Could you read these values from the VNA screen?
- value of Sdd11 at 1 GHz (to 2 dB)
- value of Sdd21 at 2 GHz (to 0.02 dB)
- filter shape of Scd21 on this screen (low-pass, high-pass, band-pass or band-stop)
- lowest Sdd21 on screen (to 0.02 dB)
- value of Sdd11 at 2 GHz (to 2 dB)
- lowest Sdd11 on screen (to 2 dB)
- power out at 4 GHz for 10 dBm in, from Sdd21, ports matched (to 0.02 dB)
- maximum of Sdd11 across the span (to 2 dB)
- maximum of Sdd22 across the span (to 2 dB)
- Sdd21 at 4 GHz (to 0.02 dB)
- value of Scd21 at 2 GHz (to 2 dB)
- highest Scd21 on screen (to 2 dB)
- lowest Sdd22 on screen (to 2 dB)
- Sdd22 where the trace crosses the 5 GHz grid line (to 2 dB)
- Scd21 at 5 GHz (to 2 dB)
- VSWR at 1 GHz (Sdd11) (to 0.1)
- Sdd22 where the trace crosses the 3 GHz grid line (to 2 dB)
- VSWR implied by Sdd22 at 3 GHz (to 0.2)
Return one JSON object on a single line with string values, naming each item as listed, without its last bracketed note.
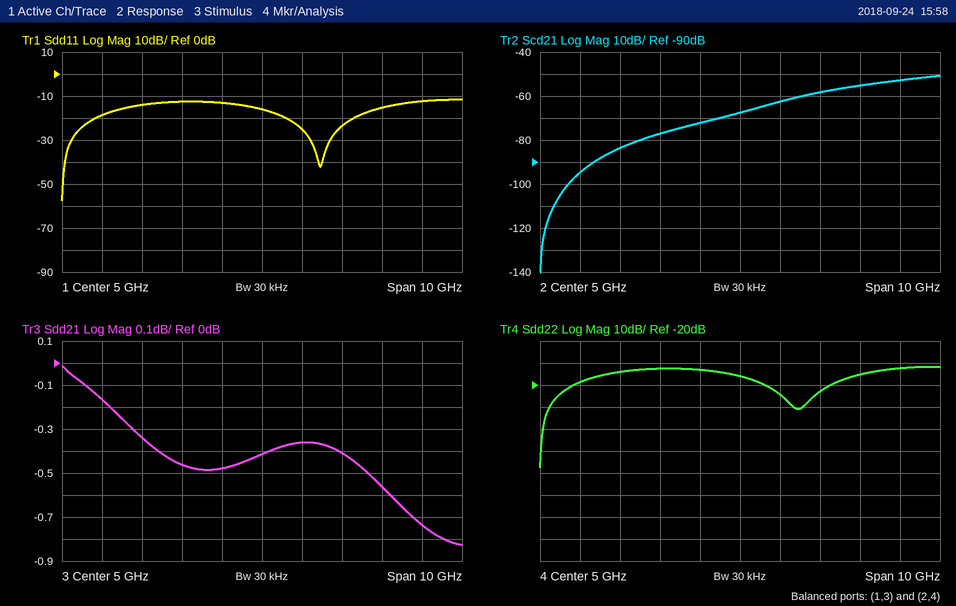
{"value of Sdd11 at 1 GHz": "-18 dB", "value of Sdd21 at 2 GHz": "-0.34 dB", "filter shape of Scd21 on this screen": "high-pass", "lowest Sdd21 on screen": "-0.82 dB", "value of Sdd11 at 2 GHz": "-14 dB", "lowest Sdd11 on screen": "-58 dB", "power out at 4 GHz for 10 dBm in, from Sdd21, ports matched": "9.52 dBm", "maximum of Sdd11 across the span": "-12 dB", "maximum of Sdd22 across the span": "-12 dB", "Sdd21 at 4 GHz": "-0.48 dB", "value of Scd21 at 2 GHz": "-84 dB", "highest Scd21 on screen": "-50 dB", "lowest Sdd22 on screen": "-58 dB", "Sdd22 where the trace crosses the 5 GHz grid line": "-16 dB", "Scd21 at 5 GHz": "-68 dB", "VSWR at 1 GHz (Sdd11)": "1.3", "Sdd22 where the trace crosses the 3 GHz grid line": "-12 dB", "VSWR implied by Sdd22 at 3 GHz": "1.6"}
